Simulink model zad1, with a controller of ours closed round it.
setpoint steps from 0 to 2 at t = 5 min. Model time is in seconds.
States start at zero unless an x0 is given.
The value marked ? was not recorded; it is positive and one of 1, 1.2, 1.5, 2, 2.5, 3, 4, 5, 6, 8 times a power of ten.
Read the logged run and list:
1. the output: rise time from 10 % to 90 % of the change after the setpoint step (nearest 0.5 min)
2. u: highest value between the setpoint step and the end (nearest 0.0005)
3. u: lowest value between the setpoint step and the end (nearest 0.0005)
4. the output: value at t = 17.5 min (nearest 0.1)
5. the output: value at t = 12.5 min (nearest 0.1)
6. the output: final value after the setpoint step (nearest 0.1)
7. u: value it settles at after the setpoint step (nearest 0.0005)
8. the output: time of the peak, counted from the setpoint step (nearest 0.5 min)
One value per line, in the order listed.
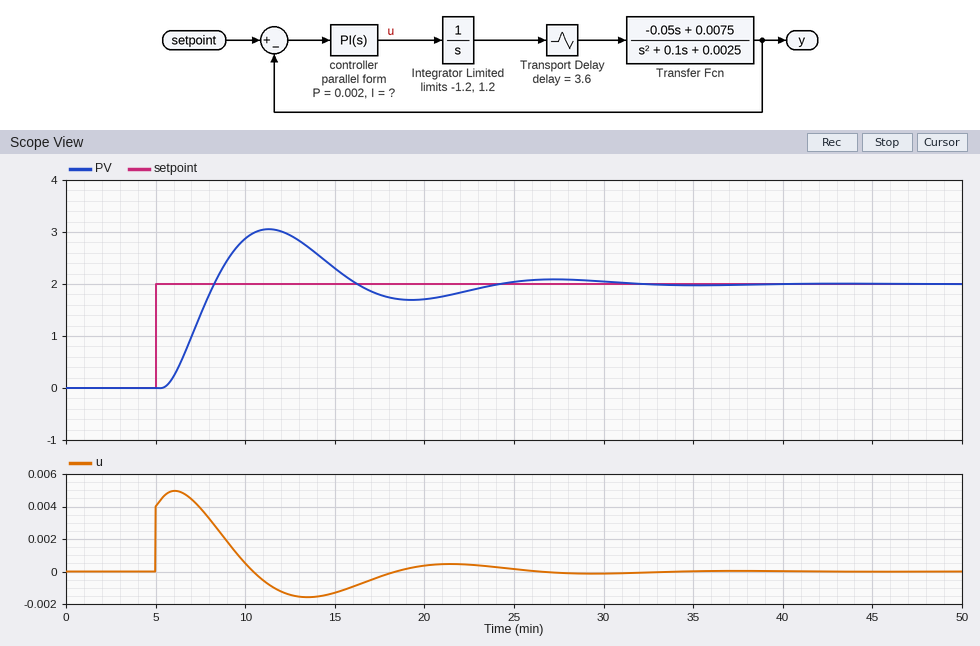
2.0 min
0.0050
-0.0015
1.8
2.9
2.0
0.0000
6.5 min
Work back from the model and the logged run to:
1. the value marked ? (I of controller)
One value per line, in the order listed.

1.2e-05
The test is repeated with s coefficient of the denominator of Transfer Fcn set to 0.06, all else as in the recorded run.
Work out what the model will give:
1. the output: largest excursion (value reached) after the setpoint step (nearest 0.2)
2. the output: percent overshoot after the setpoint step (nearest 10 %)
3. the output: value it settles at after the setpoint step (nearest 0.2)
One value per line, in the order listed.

2.8
40 %
2.0
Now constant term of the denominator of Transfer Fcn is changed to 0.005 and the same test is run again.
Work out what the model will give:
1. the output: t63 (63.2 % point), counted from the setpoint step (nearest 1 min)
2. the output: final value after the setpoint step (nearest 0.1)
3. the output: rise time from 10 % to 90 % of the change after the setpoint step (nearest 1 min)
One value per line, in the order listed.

3 min
1.8
3 min
